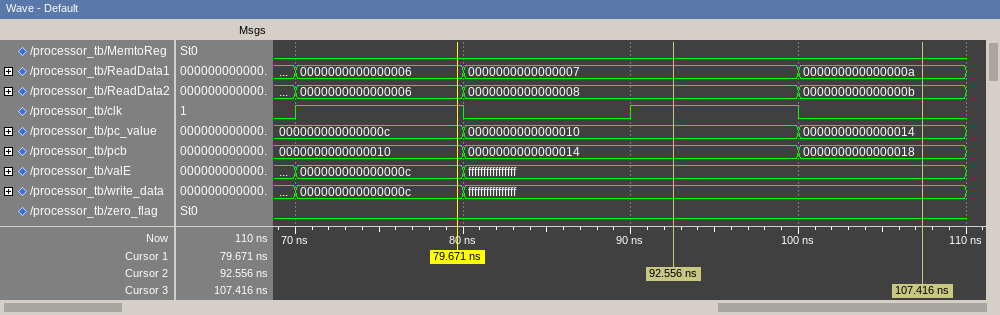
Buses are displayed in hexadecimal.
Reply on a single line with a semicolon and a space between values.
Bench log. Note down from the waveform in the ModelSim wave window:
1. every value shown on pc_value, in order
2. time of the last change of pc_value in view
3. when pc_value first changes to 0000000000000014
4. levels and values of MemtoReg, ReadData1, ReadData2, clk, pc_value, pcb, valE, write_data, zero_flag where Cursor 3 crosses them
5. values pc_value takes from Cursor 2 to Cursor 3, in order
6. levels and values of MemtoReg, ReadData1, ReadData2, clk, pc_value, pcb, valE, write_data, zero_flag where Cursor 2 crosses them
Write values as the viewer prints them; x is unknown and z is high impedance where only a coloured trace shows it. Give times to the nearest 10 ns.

000000000000000c, 0000000000000010, 0000000000000014; 100 ns; 100 ns; MemtoReg=0, ReadData1=000000000000000a, ReadData2=000000000000000b, clk=0, pc_value=0000000000000014, pcb=0000000000000018, valE=ffffffffffffffff, write_data=ffffffffffffffff, zero_flag=0; 0000000000000010, 0000000000000014; MemtoReg=0, ReadData1=0000000000000007, ReadData2=0000000000000008, clk=1, pc_value=0000000000000010, pcb=0000000000000014, valE=ffffffffffffffff, write_data=ffffffffffffffff, zero_flag=0
